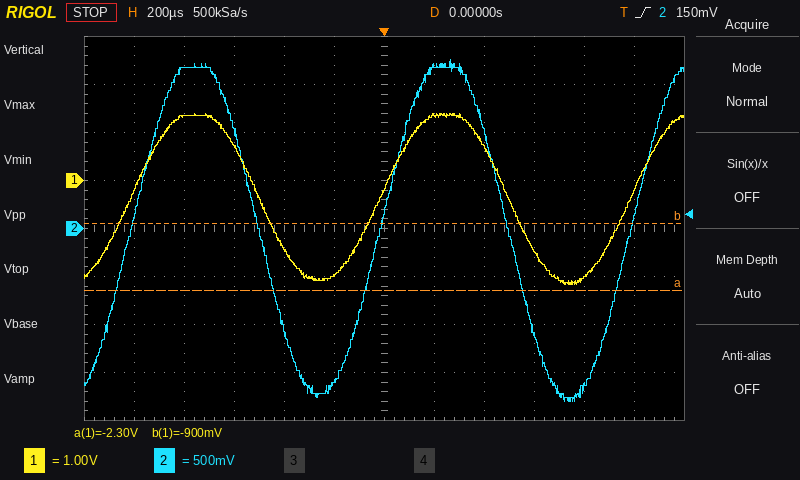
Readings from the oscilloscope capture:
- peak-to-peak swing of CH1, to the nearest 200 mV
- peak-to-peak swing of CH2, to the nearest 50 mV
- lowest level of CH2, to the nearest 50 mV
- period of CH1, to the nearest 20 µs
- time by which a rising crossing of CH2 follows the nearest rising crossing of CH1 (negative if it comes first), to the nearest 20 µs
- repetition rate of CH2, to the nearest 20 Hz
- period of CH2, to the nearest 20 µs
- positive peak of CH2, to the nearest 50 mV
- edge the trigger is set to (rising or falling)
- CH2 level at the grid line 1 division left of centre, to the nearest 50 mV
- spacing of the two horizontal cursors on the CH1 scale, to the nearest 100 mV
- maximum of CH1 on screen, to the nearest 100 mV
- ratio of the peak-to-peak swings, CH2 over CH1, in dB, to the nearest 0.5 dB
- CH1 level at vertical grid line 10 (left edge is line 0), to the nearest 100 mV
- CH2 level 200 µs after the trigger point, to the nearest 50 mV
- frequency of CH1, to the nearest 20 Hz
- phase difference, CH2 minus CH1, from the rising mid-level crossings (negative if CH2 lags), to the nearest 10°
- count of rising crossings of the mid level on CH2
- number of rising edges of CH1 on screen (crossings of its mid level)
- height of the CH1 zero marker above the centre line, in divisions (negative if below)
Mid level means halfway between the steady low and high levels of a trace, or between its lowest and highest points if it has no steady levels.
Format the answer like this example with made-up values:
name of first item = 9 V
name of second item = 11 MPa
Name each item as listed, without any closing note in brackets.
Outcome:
peak-to-peak swing of CH1, to the nearest 200 mV = 3.6 V
peak-to-peak swing of CH2, to the nearest 50 mV = 3.55 V
lowest level of CH2, to the nearest 50 mV = -1.80 V
period of CH1, to the nearest 20 µs = 1.00 ms
time by which a rising crossing of CH2 follows the nearest rising crossing of CH1 (negative if it comes first), to the nearest 20 µs = 0 µs
repetition rate of CH2, to the nearest 20 Hz = 1.00 kHz
period of CH2, to the nearest 20 µs = 1.00 ms
positive peak of CH2, to the nearest 50 mV = 1.75 V
edge the trigger is set to = rising
CH2 level at the grid line 1 division left of centre, to the nearest 50 mV = -1.60 V
spacing of the two horizontal cursors on the CH1 scale, to the nearest 100 mV = 1.4 V
maximum of CH1 on screen, to the nearest 100 mV = 1.4 V
ratio of the peak-to-peak swings, CH2 over CH1, in dB, to the nearest 0.5 dB = 0.0 dB
CH1 level at vertical grid line 10 (left edge is line 0), to the nearest 100 mV = -2.0 V
CH2 level 200 µs after the trigger point, to the nearest 50 mV = 1.70 V
frequency of CH1, to the nearest 20 Hz = 1.00 kHz
phase difference, CH2 minus CH1, from the rising mid-level crossings (negative if CH2 lags), to the nearest 10° = 0°
count of rising crossings of the mid level on CH2 = 3
number of rising edges of CH1 on screen = 3
height of the CH1 zero marker above the centre line, in divisions = +1.0 div
